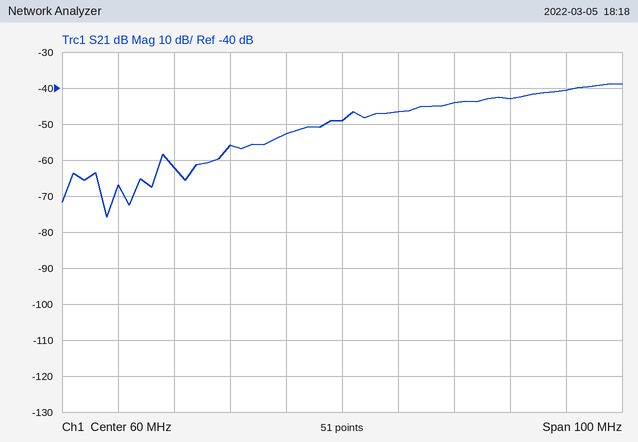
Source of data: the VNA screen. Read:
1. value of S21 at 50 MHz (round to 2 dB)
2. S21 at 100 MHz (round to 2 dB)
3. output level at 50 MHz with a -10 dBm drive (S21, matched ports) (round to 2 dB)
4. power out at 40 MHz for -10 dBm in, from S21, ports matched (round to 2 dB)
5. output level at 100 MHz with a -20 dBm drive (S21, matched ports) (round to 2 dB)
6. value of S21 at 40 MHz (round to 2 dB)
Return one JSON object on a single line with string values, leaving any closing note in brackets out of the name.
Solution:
{"value of S21 at 50 MHz": "-52 dB", "S21 at 100 MHz": "-40 dB", "output level at 50 MHz with a -10 dBm drive (S21, matched ports)": "-62 dBm", "power out at 40 MHz for -10 dBm in, from S21, ports matched": "-66 dBm", "output level at 100 MHz with a -20 dBm drive (S21, matched ports)": "-60 dBm", "value of S21 at 40 MHz": "-56 dB"}
